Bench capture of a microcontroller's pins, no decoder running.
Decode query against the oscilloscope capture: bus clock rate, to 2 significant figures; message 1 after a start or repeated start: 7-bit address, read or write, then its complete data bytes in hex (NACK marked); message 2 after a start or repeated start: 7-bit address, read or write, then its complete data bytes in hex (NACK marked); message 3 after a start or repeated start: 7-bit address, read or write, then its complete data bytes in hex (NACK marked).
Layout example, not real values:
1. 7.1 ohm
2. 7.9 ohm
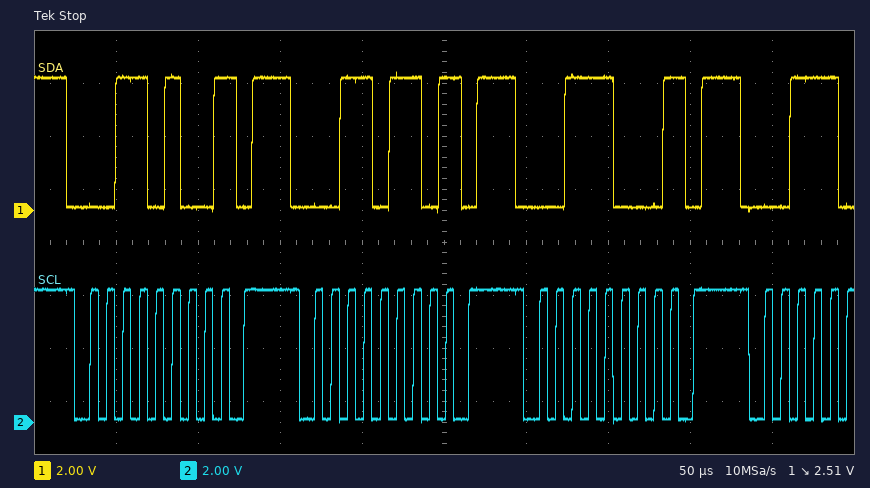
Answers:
1. 100 kHz
2. 0x1A write NACK
3. 0x1B write NACK
4. 0x1C write NACK
